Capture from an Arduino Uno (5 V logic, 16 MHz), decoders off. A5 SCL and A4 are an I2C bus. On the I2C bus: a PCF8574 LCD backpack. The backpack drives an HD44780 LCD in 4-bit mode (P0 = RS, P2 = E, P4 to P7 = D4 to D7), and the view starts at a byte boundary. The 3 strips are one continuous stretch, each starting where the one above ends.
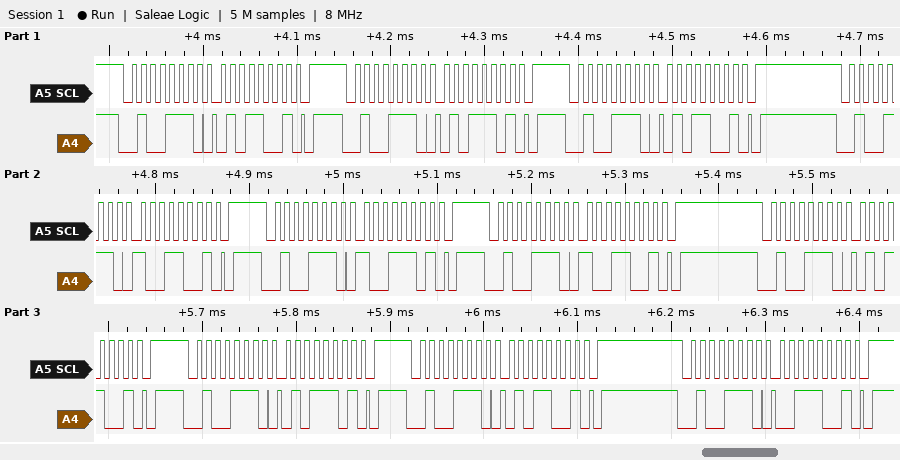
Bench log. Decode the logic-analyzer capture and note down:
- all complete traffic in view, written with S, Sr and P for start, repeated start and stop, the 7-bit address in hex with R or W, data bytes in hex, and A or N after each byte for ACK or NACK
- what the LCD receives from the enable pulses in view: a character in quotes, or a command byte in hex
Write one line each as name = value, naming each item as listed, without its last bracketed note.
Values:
all complete traffic in view, written with S, Sr and P for start, repeated start and stop, the 7-bit address in hex with R or W, data bytes in hex, and A or N after each byte for ACK or NACK = S 27W A 59 A P S 27W A 5D A P S 27W A 59 A P S 27W A 99 A P S 27W A 9D A P S 27W A 99 A P S 27W A 59 A P S 27W A 5D A P S 27W A 59 A P S 27W A 39 A P
what the LCD receives from the enable pulses in view: a character in quotes, or a command byte in hex = 'Y'
